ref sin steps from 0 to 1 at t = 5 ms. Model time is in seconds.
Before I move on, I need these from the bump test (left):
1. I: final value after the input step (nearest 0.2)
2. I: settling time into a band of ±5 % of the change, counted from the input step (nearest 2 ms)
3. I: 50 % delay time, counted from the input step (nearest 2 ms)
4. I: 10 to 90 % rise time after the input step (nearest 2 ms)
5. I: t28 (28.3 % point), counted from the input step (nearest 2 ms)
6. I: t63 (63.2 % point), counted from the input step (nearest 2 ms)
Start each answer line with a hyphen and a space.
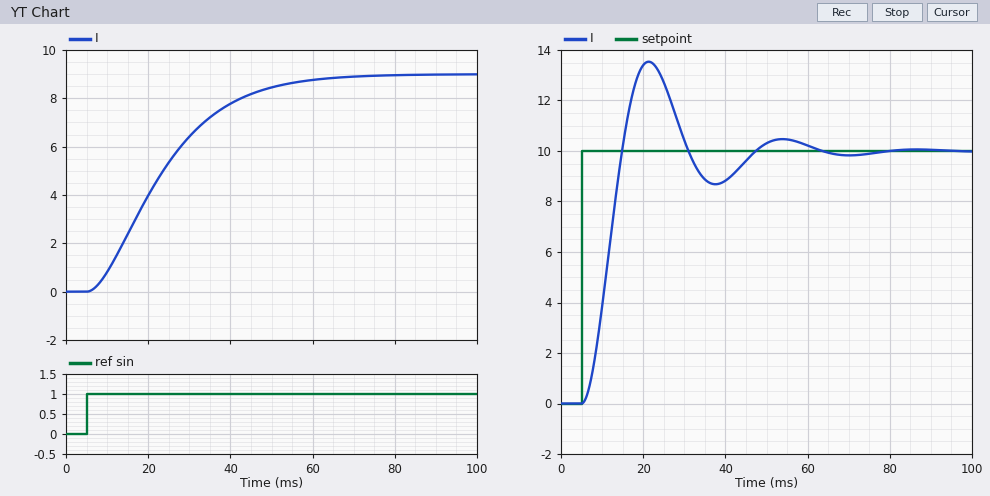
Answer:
- 9.0
- 48 ms
- 16 ms
- 34 ms
- 10 ms
- 22 ms
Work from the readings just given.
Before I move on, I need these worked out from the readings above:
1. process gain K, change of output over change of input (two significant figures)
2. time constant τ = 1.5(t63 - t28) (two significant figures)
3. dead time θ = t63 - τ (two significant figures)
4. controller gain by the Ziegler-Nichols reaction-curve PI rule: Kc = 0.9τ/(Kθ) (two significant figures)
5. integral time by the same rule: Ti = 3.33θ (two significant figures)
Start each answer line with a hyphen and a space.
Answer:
- 9.0
- 18 ms
- 4.0 ms
- 0.45
- 13 ms
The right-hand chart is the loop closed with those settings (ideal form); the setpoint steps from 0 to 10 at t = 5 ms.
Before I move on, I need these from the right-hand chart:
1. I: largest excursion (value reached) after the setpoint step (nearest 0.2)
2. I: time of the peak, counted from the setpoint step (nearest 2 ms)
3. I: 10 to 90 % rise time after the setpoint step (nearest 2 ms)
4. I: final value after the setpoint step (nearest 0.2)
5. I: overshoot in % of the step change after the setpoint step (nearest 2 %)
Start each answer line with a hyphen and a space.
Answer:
- 13.6
- 16 ms
- 6 ms
- 10.0
- 36 %
